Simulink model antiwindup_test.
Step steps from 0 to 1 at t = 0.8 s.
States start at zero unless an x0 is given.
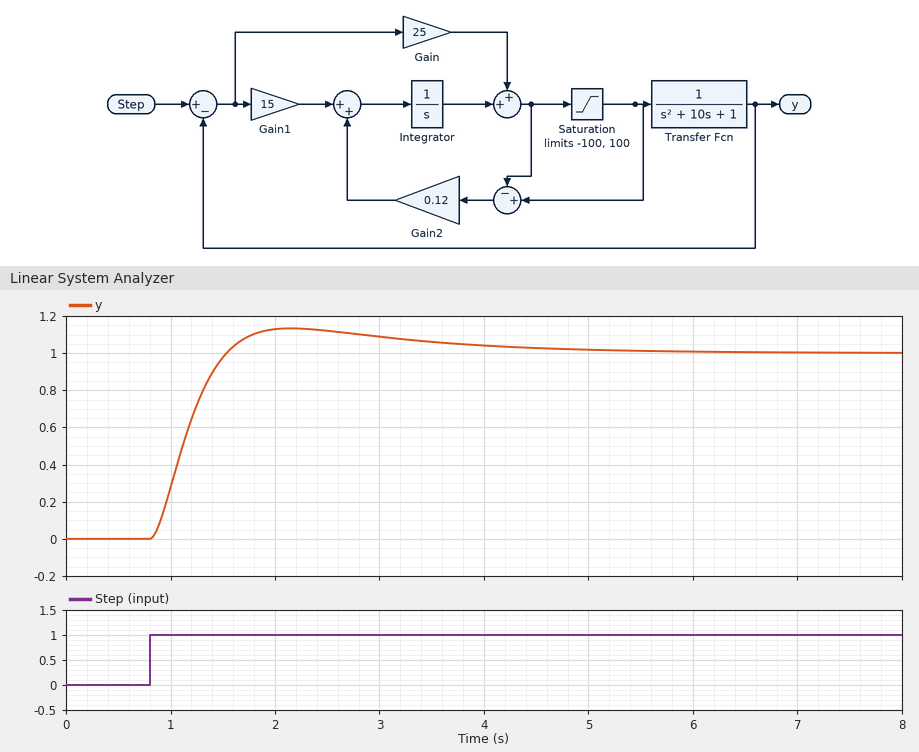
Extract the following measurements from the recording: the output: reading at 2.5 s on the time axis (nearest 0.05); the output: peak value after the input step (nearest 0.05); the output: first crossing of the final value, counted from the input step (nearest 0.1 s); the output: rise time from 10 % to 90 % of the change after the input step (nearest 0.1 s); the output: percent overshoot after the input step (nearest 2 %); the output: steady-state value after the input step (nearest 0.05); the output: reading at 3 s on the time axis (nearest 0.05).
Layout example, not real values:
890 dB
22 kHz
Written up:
1.10
1.15
0.7 s
0.5 s
14 %
1.00
1.10
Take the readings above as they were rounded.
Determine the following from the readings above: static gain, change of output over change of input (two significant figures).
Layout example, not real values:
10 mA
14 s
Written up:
1.0
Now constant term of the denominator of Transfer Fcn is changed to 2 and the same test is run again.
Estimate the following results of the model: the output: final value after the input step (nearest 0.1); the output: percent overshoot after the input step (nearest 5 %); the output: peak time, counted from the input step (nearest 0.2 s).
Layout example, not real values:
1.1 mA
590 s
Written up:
1.0
10 %
1.4 s
